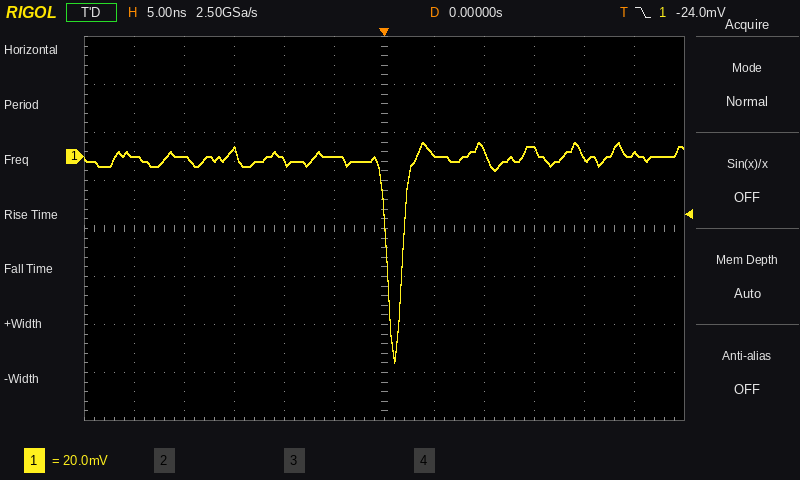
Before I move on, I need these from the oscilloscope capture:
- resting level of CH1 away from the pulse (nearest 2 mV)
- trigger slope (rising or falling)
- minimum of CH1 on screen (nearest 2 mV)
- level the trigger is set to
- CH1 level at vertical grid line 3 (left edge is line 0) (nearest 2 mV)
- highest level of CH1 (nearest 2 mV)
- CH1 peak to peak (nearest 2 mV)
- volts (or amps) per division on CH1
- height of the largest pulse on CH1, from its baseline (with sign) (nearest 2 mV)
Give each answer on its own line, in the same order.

0 mV
falling
-86 mV
-24.0 mV
2 mV
6 mV
92 mV
20 mV
-86 mV
